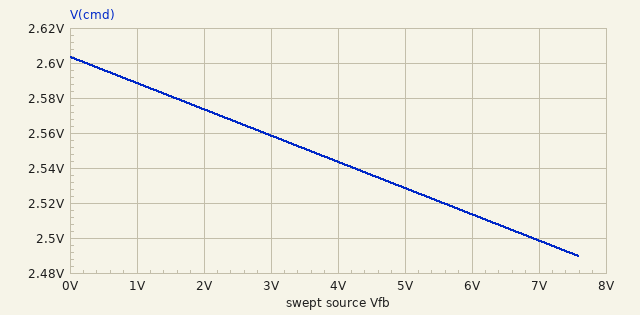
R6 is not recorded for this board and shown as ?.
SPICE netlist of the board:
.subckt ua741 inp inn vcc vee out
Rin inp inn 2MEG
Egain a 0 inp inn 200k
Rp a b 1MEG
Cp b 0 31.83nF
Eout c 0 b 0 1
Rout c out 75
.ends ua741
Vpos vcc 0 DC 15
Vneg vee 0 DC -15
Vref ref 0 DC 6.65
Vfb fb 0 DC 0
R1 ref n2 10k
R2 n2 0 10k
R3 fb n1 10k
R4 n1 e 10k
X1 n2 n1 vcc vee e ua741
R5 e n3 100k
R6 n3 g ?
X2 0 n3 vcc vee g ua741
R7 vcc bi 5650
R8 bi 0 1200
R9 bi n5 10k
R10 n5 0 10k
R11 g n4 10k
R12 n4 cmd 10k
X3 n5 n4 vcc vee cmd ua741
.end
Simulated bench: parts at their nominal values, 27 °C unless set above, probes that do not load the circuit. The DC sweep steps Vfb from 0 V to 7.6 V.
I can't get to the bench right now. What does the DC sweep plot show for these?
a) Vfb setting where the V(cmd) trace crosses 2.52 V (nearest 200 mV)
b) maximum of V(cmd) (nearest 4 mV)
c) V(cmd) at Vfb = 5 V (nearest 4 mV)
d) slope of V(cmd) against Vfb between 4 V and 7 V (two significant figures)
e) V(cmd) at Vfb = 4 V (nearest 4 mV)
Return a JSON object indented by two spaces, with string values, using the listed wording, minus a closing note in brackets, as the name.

{
  "Vfb setting where the V(cmd) trace crosses 2.52 V": "5.6 V",
  "maximum of V(cmd)": "2.604 V",
  "V(cmd) at Vfb = 5 V": "2.528 V",
  "slope of V(cmd) against Vfb between 4 V and 7 V": "-0.015 V/V",
  "V(cmd) at Vfb = 4 V": "2.544 V"
}
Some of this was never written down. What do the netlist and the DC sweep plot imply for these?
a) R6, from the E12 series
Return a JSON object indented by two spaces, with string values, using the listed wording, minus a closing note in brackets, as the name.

{
  "R6, from the E12 series": "1.5 kΩ"
}
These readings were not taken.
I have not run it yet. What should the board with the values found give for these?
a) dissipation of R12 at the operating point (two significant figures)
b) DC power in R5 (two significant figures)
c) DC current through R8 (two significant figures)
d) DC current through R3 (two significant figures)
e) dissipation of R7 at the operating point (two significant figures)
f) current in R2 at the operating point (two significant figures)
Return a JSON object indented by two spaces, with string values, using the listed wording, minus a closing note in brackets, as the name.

{
  "dissipation of R12 at the operating point": "180 µW",
  "DC power in R5": "440 µW",
  "DC current through R8": "2.1 mA",
  "DC current through R3": "330 µA",
  "dissipation of R7 at the operating point": "28 mW",
  "current in R2 at the operating point": "330 µA"
}
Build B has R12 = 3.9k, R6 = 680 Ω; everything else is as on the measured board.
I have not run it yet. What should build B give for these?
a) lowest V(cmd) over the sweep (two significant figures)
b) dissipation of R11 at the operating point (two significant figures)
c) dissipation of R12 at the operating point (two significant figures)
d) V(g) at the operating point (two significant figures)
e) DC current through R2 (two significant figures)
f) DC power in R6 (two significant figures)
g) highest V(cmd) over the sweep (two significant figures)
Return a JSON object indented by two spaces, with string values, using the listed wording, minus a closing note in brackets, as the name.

{
  "lowest V(cmd) over the sweep": "1.7 V",
  "dissipation of R11 at the operating point": "170 µW",
  "dissipation of R12 at the operating point": "66 µW",
  "V(g) at the operating point": "-45 mV",
  "DC current through R2": "330 µA",
  "DC power in R6": "3.0 µW",
  "highest V(cmd) over the sweep": "1.8 V"
}
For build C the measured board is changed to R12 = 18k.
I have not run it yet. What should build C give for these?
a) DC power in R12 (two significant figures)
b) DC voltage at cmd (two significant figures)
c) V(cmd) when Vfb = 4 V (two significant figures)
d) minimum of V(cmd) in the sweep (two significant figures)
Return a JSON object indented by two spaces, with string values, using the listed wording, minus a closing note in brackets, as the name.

{
  "DC power in R12": "330 µW",
  "DC voltage at cmd": "3.7 V",
  "V(cmd) when Vfb = 4 V": "3.6 V",
  "minimum of V(cmd) in the sweep": "3.5 V"
}
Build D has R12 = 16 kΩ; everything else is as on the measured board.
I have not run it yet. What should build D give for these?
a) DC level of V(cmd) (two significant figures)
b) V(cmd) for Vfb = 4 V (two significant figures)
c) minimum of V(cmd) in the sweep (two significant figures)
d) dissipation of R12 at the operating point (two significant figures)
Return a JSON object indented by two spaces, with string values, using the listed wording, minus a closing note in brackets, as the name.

{
  "DC level of V(cmd)": "3.4 V",
  "V(cmd) for Vfb = 4 V": "3.3 V",
  "minimum of V(cmd) in the sweep": "3.2 V",
  "dissipation of R12 at the operating point": "290 µW"
}
